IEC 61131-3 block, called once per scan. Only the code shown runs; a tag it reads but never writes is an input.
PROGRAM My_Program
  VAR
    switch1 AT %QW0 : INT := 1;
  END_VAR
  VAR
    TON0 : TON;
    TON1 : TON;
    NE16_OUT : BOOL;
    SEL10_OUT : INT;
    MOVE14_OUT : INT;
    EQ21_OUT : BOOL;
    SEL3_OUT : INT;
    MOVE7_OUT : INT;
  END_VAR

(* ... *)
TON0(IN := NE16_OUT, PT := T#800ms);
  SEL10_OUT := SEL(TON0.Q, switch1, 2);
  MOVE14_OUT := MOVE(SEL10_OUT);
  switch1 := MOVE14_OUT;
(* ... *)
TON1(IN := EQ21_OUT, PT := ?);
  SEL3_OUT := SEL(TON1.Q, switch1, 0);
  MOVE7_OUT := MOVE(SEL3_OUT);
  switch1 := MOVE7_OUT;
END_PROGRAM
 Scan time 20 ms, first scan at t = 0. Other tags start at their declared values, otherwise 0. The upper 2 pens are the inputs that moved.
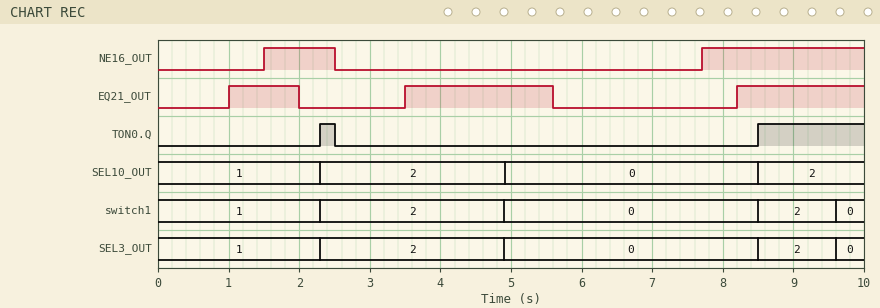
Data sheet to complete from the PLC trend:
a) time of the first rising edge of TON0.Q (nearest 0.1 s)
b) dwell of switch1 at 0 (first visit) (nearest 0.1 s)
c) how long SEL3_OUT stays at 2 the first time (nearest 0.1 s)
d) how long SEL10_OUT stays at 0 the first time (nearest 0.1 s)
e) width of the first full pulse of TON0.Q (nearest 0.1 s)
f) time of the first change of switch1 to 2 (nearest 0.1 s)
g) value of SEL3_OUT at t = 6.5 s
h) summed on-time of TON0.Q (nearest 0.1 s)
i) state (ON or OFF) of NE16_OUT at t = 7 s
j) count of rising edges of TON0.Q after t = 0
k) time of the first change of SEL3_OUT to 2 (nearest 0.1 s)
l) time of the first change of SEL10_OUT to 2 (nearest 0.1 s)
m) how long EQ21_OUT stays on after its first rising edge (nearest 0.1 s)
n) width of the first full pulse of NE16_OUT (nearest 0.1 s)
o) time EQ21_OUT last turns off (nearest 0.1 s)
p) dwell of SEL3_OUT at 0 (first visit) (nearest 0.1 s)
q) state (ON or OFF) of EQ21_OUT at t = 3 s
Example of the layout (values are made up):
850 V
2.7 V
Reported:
2.3 s
3.6 s
2.6 s
3.6 s
0.2 s
2.3 s
0
1.7 s
OFF
2
2.3 s
2.3 s
1.0 s
1.0 s
5.6 s
3.6 s
OFF
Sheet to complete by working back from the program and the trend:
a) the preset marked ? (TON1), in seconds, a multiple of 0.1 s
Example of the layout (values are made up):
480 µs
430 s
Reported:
1.4 s
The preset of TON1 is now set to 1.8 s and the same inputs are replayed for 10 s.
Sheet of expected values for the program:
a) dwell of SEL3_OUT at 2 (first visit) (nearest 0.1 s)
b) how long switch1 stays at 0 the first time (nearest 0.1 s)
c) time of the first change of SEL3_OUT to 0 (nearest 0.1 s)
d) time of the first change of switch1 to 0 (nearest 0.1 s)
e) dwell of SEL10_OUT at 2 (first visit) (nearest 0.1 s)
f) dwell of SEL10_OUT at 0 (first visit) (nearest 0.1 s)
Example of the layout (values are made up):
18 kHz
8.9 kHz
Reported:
3.0 s
3.2 s
5.3 s
5.3 s
3.0 s
3.2 s
